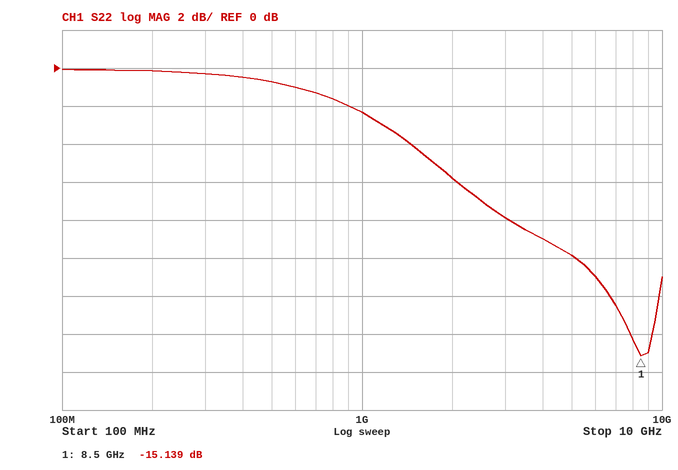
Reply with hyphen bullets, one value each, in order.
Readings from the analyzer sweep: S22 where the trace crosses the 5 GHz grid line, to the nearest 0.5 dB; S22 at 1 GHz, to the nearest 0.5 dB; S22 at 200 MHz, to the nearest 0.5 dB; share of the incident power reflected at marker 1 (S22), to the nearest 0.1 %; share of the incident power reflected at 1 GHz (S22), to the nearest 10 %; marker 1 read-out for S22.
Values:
- -10.0 dB
- -2.5 dB
- 0.0 dB
- 3.1 %
- 60 %
- -15.139 dB
